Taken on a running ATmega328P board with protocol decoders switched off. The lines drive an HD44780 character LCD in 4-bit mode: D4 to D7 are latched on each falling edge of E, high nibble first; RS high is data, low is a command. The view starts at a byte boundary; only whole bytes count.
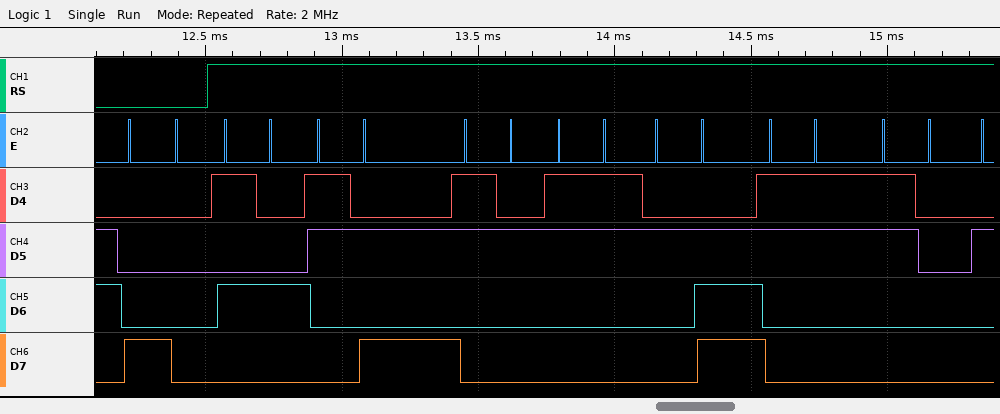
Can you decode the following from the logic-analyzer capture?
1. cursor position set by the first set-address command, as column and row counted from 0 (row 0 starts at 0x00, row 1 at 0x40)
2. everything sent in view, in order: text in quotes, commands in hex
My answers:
column 0, row 0
0x80 "T:23.30"
